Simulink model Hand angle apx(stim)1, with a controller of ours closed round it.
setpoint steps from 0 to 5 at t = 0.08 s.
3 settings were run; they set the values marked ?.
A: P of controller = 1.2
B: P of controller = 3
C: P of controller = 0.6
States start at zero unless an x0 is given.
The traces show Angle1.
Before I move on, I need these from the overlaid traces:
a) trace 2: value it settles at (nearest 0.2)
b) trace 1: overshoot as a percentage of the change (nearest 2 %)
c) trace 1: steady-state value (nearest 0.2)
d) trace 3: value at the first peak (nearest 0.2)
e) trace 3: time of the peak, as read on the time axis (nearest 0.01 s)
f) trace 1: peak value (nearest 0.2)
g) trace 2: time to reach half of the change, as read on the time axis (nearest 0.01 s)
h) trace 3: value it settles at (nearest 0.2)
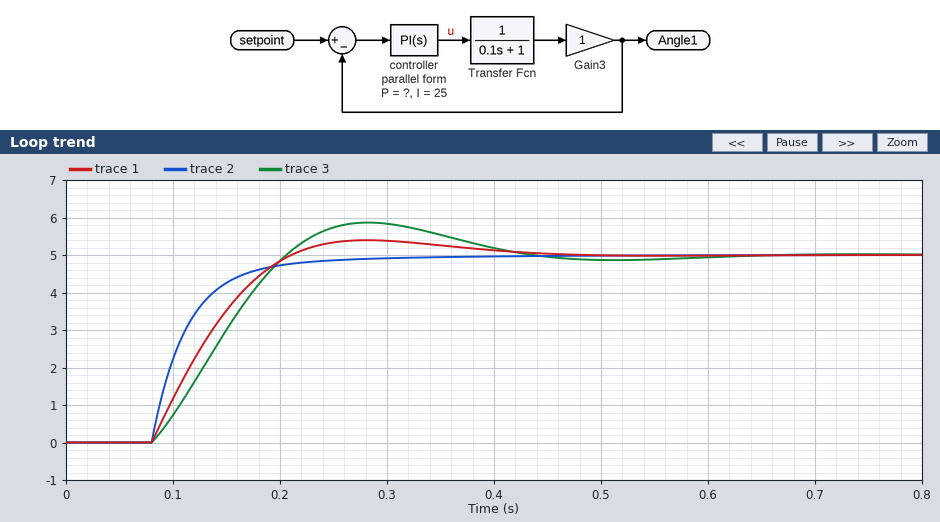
5.0
8 %
5.0
5.8
0.28 s
5.4
0.10 s
5.0
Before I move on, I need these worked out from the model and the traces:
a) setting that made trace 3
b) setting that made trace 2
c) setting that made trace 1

C
B
A
